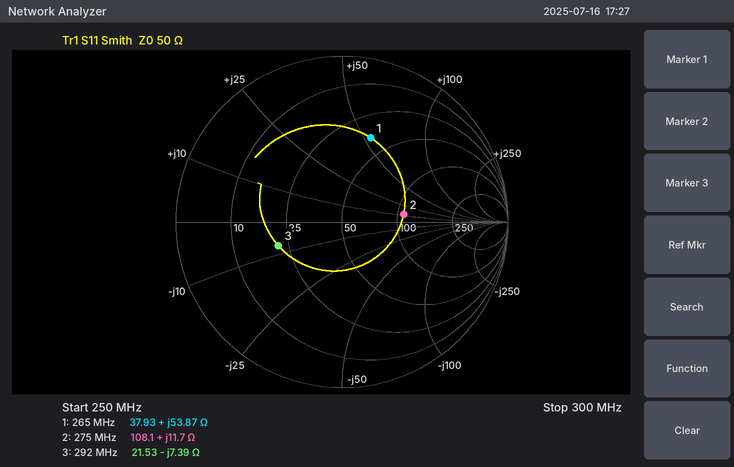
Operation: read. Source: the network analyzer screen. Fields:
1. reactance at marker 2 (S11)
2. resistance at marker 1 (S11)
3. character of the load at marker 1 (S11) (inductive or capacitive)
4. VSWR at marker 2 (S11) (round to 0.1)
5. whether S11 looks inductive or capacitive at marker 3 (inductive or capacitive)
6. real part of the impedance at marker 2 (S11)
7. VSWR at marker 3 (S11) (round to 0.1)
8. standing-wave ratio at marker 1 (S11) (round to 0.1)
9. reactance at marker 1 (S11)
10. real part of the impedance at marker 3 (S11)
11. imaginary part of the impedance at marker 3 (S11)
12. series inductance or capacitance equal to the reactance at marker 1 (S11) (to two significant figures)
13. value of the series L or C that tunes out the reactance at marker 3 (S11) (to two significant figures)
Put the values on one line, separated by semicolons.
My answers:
+11.7 Ω; 37.93 Ω; inductive; 2.2; capacitive; 108.1 Ω; 2.4; 3.3; +53.87 Ω; 21.53 Ω; -7.39 Ω; 32 nH; 4.0 nH
